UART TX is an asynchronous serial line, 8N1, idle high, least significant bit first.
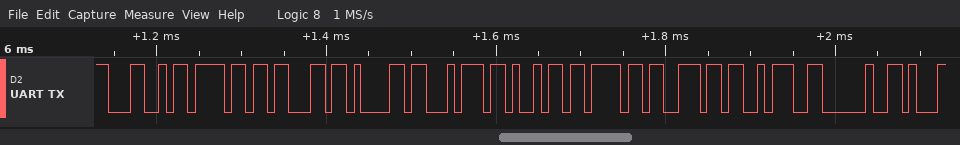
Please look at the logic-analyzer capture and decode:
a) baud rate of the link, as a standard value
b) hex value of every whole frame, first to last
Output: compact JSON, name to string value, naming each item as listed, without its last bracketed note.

{"baud rate of the link, as a standard value": "115200 baud", "hex value of every whole frame, first to last": "0x4C 0x6F 0x63 0x61 0x74 0x69 0x6F 0x6E 0x3A 0x20"}
